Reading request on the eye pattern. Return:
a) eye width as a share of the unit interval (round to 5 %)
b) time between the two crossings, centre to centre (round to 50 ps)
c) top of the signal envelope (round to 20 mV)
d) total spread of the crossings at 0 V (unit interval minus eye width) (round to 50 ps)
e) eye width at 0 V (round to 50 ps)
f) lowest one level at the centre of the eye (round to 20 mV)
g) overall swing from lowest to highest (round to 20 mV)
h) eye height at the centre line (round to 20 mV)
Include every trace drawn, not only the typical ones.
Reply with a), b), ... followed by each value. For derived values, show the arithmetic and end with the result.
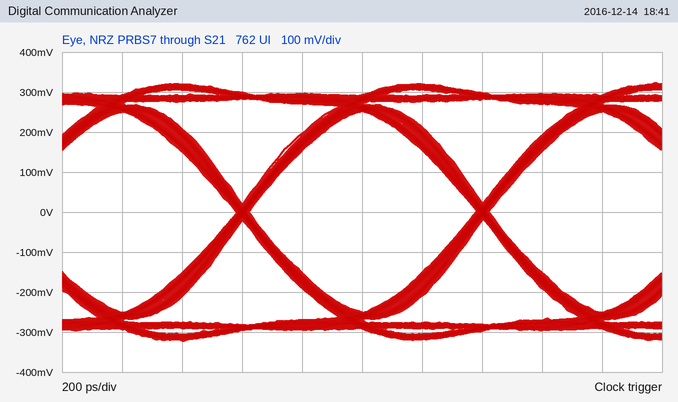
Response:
a) 750 ps / 800 ps ≈ 93.7 %, so 95 % to the nearest 5 %
b) 800 ps
c) 320 mV
d) 50 ps
e) 750 ps
f) 260 mV
g) 640 mV
h) 500 mV
